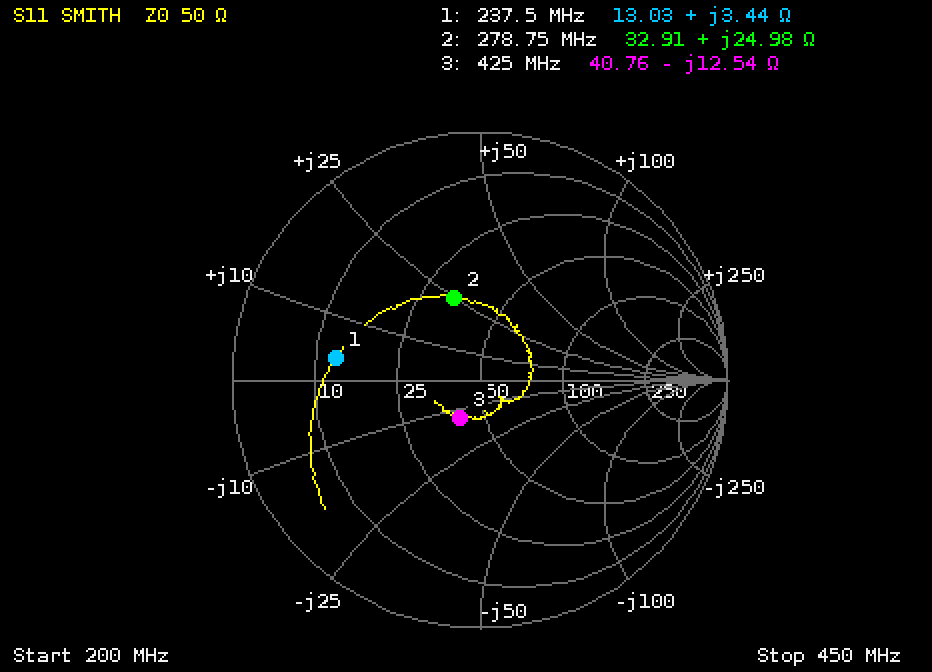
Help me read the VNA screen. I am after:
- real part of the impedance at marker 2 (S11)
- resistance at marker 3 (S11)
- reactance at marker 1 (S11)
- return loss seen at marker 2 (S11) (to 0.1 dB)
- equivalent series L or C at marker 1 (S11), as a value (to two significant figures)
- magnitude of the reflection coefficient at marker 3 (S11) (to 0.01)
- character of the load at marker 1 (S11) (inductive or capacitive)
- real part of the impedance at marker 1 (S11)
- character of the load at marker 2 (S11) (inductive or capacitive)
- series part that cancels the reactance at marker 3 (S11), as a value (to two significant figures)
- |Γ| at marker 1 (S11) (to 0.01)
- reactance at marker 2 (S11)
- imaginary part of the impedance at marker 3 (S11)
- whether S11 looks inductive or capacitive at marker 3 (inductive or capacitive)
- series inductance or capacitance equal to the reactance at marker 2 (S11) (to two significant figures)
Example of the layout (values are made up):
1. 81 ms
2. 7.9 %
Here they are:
1. 32.91 Ω
2. 40.76 Ω
3. +3.44 Ω
4. 9.1 dB
5. 2.3 nH
6. 0.17
7. inductive
8. 13.03 Ω
9. inductive
10. 4.7 nH
11. 0.59
12. +24.98 Ω
13. -12.54 Ω
14. capacitive
15. 14 nH
